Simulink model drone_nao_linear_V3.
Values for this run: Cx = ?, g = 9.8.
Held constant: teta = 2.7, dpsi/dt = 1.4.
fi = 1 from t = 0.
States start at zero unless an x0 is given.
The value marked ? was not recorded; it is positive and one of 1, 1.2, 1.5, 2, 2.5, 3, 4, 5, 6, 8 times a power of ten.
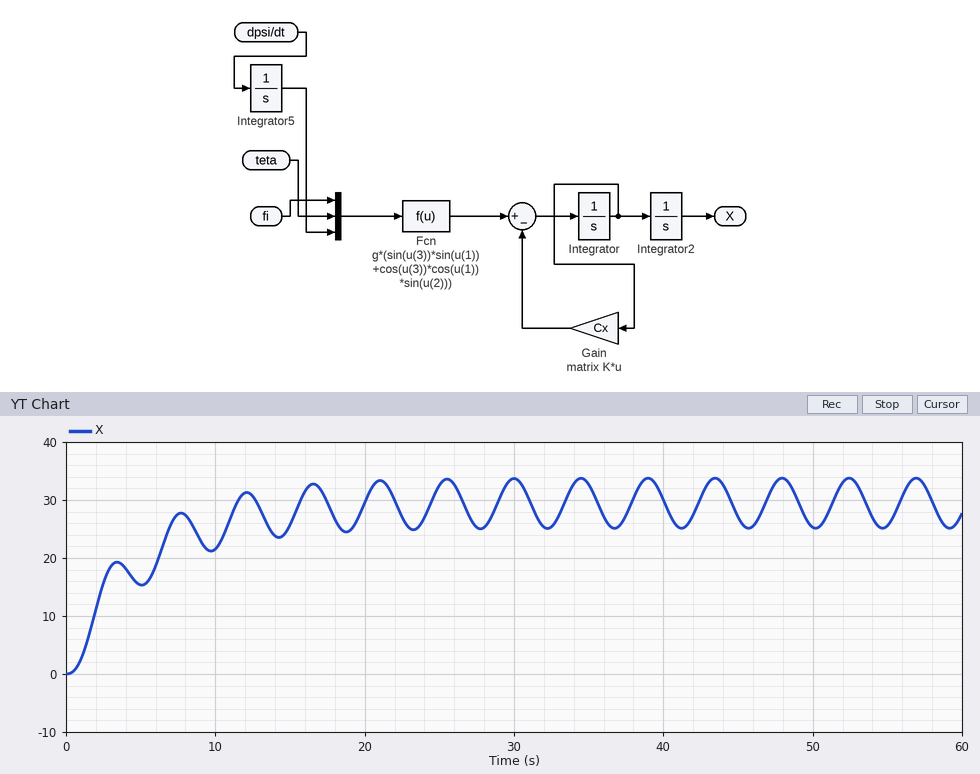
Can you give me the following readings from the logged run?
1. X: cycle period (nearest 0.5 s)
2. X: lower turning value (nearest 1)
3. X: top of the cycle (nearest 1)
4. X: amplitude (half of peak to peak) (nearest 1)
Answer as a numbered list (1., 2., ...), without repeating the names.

1. 4.5 s
2. 25
3. 34
4. 4
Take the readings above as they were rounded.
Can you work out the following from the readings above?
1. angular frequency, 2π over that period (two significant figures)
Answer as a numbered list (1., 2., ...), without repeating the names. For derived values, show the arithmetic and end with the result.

1. 2π / 4.5 = 1.4 rad/s
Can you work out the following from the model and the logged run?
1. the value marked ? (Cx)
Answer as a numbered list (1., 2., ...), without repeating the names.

1. 0.2
